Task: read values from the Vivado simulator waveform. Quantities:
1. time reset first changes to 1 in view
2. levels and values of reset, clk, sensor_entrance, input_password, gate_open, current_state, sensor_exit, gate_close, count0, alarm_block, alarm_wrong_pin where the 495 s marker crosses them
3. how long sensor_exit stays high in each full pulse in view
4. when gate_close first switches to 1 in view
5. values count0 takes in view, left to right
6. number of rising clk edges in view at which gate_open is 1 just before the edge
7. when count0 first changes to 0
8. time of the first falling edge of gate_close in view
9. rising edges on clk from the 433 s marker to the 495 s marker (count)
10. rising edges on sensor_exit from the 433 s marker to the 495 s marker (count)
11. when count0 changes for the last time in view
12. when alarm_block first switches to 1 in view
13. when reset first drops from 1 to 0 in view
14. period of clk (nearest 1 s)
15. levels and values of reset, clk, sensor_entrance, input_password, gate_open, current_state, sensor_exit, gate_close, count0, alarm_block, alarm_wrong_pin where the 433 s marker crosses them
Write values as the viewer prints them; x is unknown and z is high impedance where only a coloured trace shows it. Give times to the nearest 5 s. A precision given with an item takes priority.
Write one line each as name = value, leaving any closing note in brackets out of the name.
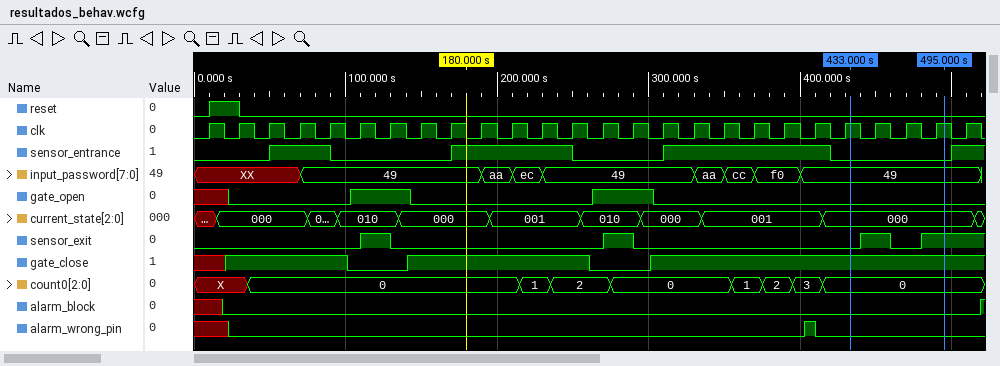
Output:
time reset first changes to 1 in view = 10 s
levels and values of reset, clk, sensor_entrance, input_password, gate_open, current_state, sensor_exit, gate_close, count0, alarm_block, alarm_wrong_pin where the 495 s marker crosses them = reset=0, clk=1, sensor_entrance=0, input_password=49, gate_open=0, current_state=000, sensor_exit=1, gate_close=1, count0=0, alarm_block=0, alarm_wrong_pin=0
how long sensor_exit stays high in each full pulse in view = 20 s, 20 s, 20 s
when gate_close first switches to 1 in view = 20 s
values count0 takes in view, left to right = X, 0, 1, 2, 0, 1, 2, 3, 0
number of rising clk edges in view at which gate_open is 1 just before the edge = 4
when count0 first changes to 0 = 35 s
time of the first falling edge of gate_close in view = 100 s
rising edges on clk from the 433 s marker to the 495 s marker = 3
rising edges on sensor_exit from the 433 s marker to the 495 s marker = 2
when count0 changes for the last time in view = 415 s
when alarm_block first switches to 1 in view = 520 s
when reset first drops from 1 to 0 in view = 30 s
period of clk = 20 s
levels and values of reset, clk, sensor_entrance, input_password, gate_open, current_state, sensor_exit, gate_close, count0, alarm_block, alarm_wrong_pin where the 433 s marker crosses them = reset=0, clk=1, sensor_entrance=0, input_password=49, gate_open=0, current_state=000, sensor_exit=0, gate_close=1, count0=0, alarm_block=0, alarm_wrong_pin=0
